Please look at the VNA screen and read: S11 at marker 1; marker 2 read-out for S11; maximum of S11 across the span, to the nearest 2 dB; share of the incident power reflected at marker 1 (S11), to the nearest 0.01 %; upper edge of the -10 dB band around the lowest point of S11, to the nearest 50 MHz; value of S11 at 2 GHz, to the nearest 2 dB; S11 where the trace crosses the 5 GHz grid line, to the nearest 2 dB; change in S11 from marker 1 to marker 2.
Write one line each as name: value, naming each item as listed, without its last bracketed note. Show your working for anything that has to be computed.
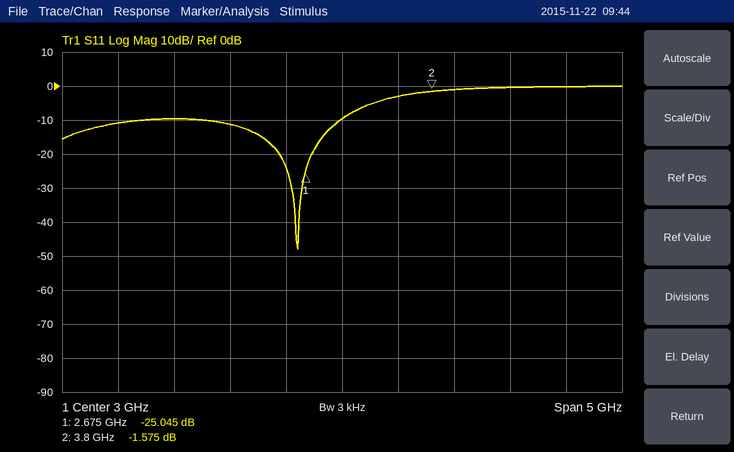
S11 at marker 1: -25.045 dB
marker 2 read-out for S11: -1.575 dB
maximum of S11 across the span, to the nearest 2 dB: 0 dB
share of the incident power reflected at marker 1 (S11), to the nearest 0.01 %: 10^(-25.045/10) ≈ 0.31 %
upper edge of the -10 dB band around the lowest point of S11, to the nearest 50 MHz: 3.00 GHz
value of S11 at 2 GHz, to the nearest 2 dB: -12 dB
S11 where the trace crosses the 5 GHz grid line, to the nearest 2 dB: 0 dB
change in S11 from marker 1 to marker 2: -1.575 − (-25.045) = 23.470 dB
